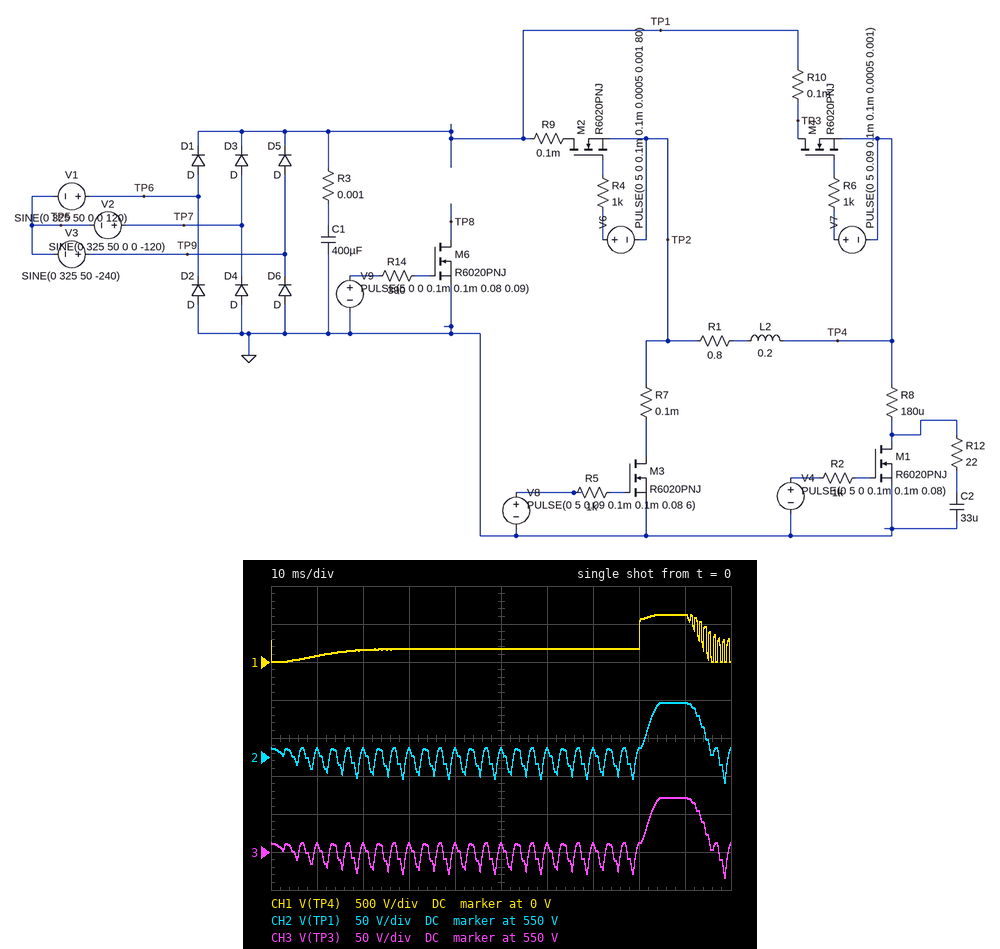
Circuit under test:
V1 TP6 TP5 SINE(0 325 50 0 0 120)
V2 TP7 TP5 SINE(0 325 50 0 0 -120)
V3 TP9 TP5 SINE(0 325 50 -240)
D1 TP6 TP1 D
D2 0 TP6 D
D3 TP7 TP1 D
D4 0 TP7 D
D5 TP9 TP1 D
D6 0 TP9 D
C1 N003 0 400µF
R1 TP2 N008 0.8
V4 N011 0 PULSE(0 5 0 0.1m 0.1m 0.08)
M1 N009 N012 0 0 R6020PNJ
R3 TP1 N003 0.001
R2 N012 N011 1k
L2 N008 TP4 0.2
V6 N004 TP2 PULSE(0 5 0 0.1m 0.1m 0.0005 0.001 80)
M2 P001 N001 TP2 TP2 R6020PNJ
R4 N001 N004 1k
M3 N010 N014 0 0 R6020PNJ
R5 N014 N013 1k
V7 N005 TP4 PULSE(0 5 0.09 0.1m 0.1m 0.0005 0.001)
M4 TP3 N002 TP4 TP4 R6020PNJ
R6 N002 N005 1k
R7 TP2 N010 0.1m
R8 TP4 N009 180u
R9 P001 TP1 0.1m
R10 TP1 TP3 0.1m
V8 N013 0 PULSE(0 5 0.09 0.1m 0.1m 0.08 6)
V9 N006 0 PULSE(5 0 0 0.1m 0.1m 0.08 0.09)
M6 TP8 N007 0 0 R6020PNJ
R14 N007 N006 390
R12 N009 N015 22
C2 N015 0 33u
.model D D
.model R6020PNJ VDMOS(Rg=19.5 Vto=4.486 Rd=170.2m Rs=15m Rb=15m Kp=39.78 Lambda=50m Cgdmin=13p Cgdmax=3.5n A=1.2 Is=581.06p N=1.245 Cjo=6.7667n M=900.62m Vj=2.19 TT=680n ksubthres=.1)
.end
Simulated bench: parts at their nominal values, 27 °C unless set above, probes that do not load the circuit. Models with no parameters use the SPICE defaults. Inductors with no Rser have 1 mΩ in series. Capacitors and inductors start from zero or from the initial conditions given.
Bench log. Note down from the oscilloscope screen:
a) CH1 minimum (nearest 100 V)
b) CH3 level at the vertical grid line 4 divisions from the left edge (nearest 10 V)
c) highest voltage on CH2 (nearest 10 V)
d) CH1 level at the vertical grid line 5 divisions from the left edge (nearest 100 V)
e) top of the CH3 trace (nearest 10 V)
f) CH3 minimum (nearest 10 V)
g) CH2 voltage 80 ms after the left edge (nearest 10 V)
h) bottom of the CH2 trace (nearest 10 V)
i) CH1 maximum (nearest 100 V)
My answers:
0 V
560 V
620 V
200 V
620 V
520 V
560 V
520 V
600 V
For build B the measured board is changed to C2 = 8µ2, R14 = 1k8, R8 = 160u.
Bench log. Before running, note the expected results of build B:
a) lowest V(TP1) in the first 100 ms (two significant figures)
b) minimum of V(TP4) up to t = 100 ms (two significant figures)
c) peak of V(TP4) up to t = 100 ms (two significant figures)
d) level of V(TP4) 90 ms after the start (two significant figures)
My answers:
520 V
-920 mV
650 V
640 V
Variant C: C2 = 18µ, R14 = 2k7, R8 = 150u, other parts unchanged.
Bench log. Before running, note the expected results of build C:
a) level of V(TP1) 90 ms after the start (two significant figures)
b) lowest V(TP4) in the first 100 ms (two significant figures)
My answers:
640 V
-880 mV
